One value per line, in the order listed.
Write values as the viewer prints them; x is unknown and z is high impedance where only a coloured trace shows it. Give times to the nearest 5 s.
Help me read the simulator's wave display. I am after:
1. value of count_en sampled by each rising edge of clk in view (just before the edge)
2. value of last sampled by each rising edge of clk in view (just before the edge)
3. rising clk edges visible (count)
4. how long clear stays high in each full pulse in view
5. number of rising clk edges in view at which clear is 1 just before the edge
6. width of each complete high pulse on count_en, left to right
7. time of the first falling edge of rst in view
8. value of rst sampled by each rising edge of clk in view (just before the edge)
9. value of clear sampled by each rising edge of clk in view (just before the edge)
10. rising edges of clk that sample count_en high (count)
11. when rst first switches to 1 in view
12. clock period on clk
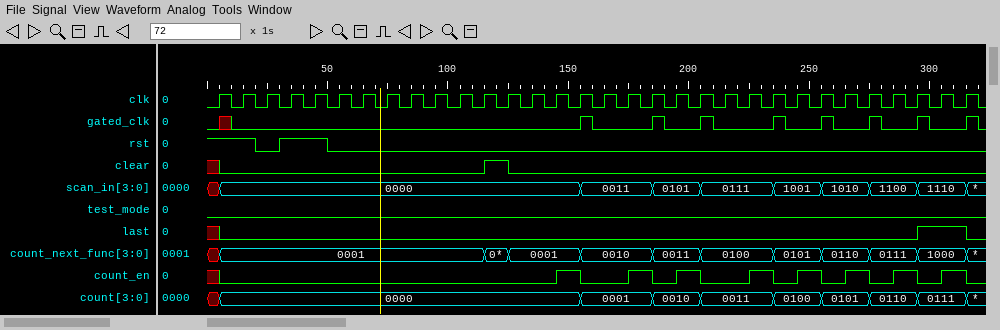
x 0 0 0 0 0 0 0 0 0 0 0 0 0 0 1 0 0 1 0 1 0 0 1 0 1 0 1 0 1 0 1
x 0 0 0 0 0 0 0 0 0 0 0 0 0 0 0 0 0 0 0 0 0 0 0 0 0 0 0 0 0 1 1
32
10 s
1
10 s, 10 s, 10 s, 10 s, 10 s, 10 s, 10 s, 10 s
20 s
1 1 0 1 1 0 0 0 0 0 0 0 0 0 0 0 0 0 0 0 0 0 0 0 0 0 0 0 0 0 0 0
x 0 0 0 0 0 0 0 0 0 0 0 1 0 0 0 0 0 0 0 0 0 0 0 0 0 0 0 0 0 0 0
8
30 s
10 s
